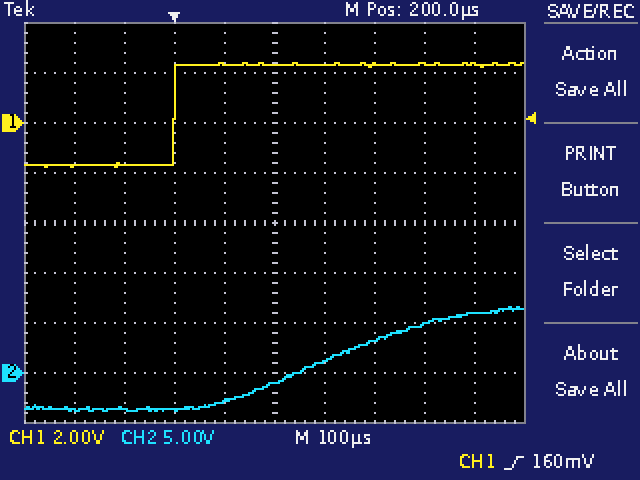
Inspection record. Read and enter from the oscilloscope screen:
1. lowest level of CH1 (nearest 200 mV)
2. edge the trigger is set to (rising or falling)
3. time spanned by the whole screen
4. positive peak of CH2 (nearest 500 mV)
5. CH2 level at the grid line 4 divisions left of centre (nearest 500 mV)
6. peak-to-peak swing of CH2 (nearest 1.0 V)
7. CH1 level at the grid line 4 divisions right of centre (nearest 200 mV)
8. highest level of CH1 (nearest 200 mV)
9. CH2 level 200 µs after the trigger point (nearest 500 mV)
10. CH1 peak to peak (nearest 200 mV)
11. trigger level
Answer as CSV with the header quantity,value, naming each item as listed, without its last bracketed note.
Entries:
quantity,value
lowest level of CH1,-1.8 V
edge the trigger is set to,rising
time spanned by the whole screen,1 ms
positive peak of CH2,6.5 V
CH2 level at the grid line 4 divisions left of centre,-3.5 V
peak-to-peak swing of CH2,10.0 V
CH1 level at the grid line 4 divisions right of centre,2.4 V
highest level of CH1,2.4 V
CH2 level 200 µs after the trigger point,-1.0 V
CH1 peak to peak,4.2 V
trigger level,160 mV
